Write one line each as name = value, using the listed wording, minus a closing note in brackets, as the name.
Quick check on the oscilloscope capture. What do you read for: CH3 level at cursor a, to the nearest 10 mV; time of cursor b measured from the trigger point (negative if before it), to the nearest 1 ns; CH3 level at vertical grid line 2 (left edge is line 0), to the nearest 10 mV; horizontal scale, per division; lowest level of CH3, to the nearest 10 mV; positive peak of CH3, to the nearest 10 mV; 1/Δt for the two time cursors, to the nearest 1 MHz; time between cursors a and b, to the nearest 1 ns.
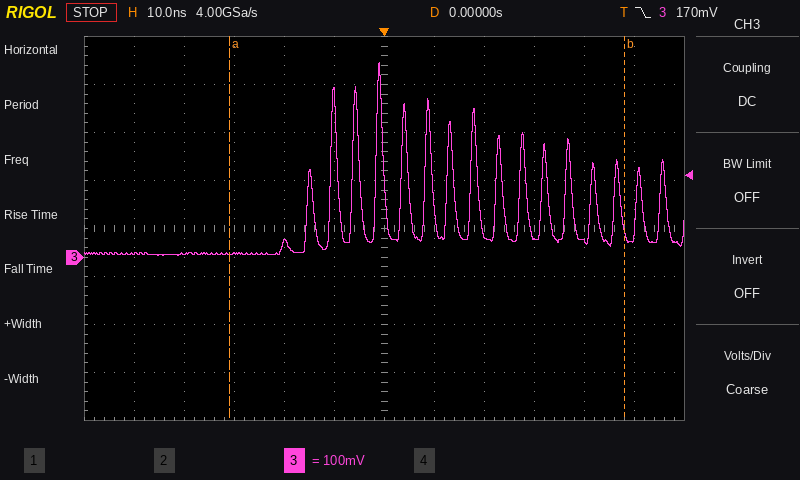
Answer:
CH3 level at cursor a, to the nearest 10 mV = 10 mV
time of cursor b measured from the trigger point (negative if before it), to the nearest 1 ns = +48 ns
CH3 level at vertical grid line 2 (left edge is line 0), to the nearest 10 mV = 10 mV
horizontal scale, per division = 10 ns
lowest level of CH3, to the nearest 10 mV = 0 mV
positive peak of CH3, to the nearest 10 mV = 410 mV
1/Δt for the two time cursors, to the nearest 1 MHz = 13 MHz
time between cursors a and b, to the nearest 1 ns = 79 ns
